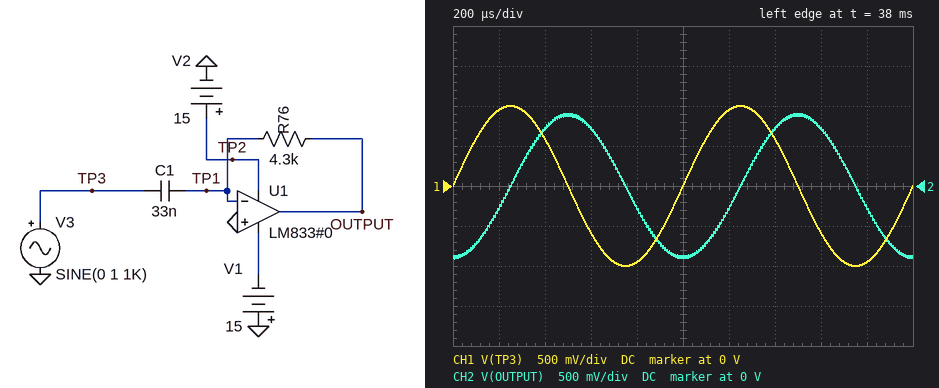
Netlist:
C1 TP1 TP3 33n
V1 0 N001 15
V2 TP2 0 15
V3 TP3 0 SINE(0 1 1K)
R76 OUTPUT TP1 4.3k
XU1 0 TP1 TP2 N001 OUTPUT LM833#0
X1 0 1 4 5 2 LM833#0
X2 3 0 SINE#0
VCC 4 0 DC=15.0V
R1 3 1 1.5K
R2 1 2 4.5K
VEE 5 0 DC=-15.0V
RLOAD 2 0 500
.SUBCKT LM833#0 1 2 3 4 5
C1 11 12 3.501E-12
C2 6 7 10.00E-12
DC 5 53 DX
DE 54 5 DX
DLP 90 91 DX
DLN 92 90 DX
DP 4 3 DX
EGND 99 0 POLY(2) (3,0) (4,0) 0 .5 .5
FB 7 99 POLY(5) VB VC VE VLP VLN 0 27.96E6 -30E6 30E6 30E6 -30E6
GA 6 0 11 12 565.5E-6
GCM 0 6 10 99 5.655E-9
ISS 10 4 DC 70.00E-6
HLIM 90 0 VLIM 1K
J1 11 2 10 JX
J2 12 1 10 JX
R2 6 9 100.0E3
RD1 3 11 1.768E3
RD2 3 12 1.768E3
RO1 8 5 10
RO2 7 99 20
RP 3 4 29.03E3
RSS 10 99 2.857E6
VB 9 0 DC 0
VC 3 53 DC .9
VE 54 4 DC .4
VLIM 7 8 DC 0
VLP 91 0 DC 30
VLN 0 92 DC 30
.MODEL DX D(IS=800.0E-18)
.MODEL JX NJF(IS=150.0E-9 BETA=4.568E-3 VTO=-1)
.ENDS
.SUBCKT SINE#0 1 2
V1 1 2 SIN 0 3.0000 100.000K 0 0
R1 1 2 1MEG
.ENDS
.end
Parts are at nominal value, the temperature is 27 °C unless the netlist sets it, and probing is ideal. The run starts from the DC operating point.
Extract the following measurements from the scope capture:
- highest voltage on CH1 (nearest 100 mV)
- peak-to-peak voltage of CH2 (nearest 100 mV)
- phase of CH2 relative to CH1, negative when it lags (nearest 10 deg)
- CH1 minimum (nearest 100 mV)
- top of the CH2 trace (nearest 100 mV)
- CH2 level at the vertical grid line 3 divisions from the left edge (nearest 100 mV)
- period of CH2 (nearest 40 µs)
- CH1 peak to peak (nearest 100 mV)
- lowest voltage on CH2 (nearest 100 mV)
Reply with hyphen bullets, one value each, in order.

- 1.0 V
- 1.8 V
- -90 deg
- -1.0 V
- 900 mV
- 700 mV
- 1.00 ms
- 2.0 V
- -900 mV
